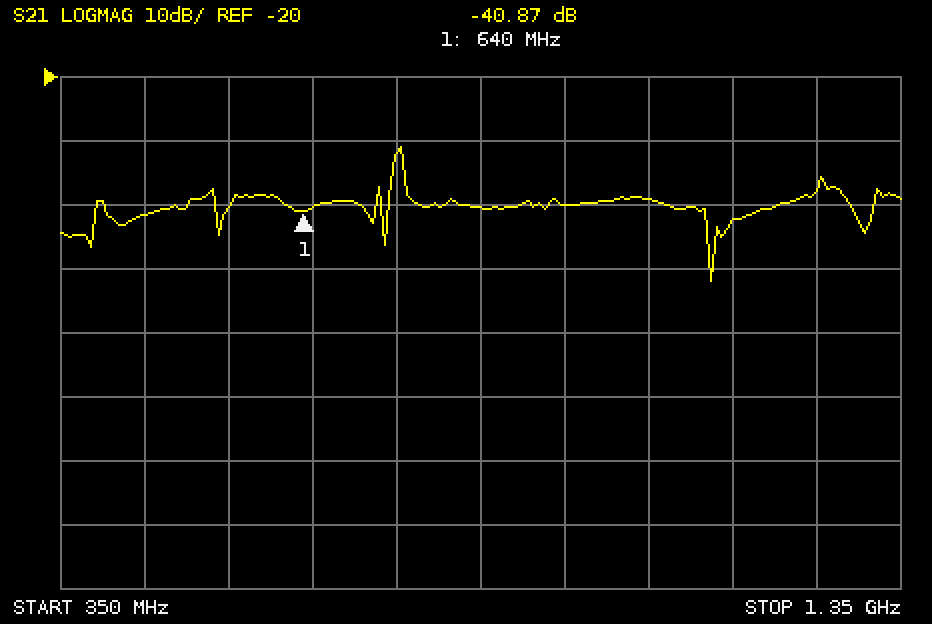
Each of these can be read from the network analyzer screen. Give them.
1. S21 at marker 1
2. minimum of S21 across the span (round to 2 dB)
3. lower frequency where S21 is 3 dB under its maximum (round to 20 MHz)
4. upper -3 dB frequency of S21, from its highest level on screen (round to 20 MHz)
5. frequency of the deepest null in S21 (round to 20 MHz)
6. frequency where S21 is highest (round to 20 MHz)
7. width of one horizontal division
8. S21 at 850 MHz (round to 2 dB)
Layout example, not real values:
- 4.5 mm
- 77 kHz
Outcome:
- -40.87 dB
- -52 dB
- 740 MHz
- 760 MHz
- 1.12 GHz
- 760 MHz
- 100 MHz
- -40 dB
